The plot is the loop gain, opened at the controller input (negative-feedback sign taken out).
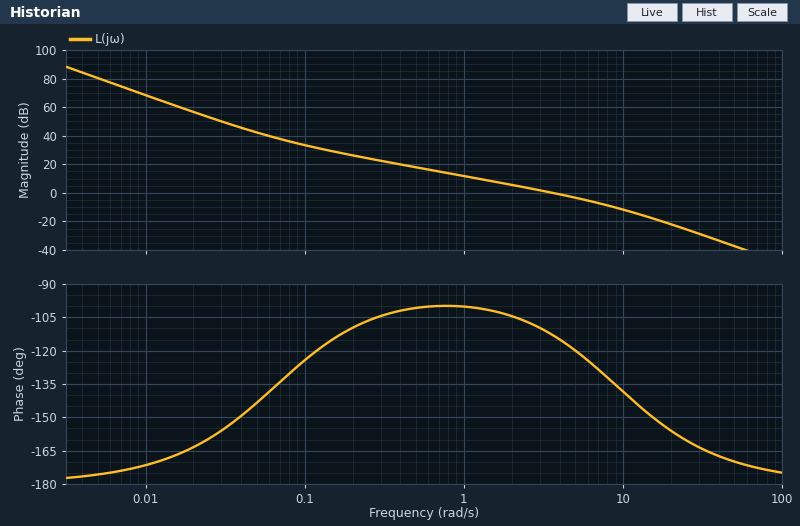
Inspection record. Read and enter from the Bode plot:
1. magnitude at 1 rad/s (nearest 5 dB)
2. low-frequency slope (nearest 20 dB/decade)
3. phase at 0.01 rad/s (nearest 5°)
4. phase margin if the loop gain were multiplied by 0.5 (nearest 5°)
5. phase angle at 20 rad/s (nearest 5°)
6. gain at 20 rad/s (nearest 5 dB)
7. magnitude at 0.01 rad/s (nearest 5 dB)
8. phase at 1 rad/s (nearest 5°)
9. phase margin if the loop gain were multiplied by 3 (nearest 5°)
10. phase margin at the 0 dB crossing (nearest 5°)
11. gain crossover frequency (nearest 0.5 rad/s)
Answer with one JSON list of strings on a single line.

["10 dB", "-40 dB/decade", "-170°", "75°", "-155°", "-20 dB", "70 dB", "-100°", "45°", "65°", "3.5 rad/s"]
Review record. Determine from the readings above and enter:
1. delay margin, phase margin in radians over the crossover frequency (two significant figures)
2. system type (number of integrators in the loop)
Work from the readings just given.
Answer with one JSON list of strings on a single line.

["0.32 s", "2"]
